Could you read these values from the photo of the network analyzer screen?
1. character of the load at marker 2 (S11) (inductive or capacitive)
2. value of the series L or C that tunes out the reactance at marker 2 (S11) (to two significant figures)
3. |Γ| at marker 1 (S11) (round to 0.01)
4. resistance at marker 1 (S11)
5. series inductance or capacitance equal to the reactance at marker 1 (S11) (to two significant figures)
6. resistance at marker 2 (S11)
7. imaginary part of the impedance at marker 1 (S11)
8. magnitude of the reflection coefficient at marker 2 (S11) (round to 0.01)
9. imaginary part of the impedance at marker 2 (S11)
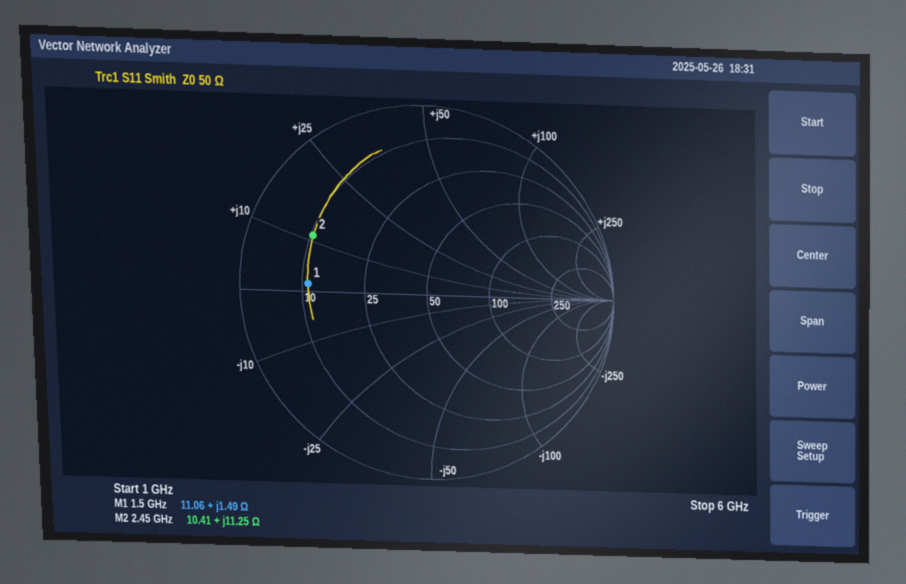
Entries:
inductive
5.8 pF
0.64
11.06 Ω
160 pH
10.41 Ω
+1.49 Ω
0.67
+11.25 Ω
